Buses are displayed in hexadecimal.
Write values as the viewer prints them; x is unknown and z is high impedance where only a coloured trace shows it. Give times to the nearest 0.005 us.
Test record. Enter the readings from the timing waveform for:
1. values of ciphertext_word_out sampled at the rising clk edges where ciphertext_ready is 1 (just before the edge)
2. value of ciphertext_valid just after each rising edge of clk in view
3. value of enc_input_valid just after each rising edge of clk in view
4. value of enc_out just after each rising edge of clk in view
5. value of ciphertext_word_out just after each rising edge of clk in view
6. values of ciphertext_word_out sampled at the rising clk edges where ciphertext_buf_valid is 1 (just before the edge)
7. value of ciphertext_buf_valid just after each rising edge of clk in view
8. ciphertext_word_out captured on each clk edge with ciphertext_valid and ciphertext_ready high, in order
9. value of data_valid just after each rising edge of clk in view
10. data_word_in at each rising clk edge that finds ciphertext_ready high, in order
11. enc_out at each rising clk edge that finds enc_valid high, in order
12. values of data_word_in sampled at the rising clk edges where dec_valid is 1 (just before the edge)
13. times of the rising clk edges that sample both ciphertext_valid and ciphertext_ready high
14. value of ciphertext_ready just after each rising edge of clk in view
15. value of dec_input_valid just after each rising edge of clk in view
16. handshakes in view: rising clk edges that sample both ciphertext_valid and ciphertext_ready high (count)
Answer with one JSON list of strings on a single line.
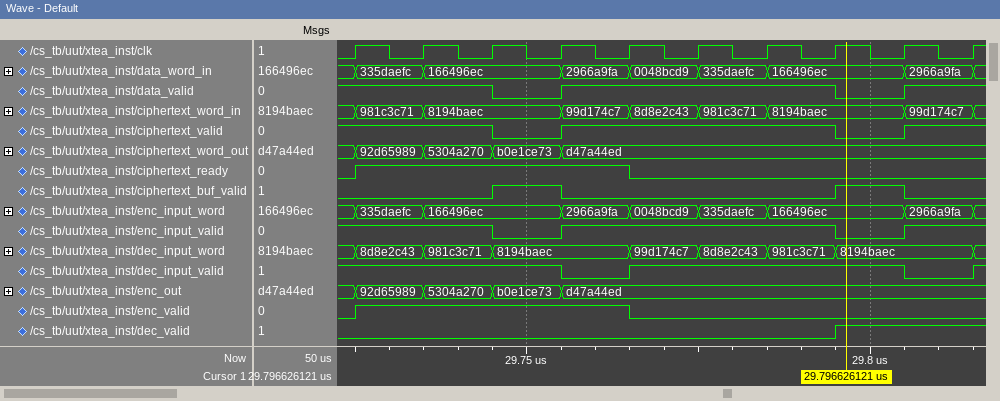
["92d65989, 5304a270, b0e1ce73, d47a44ed", "1 1 0 1 1 1 1 0 1 1", "1 1 0 1 1 1 1 0 1 1", "92d65989, 5304a270, b0e1ce73, d47a44ed, d47a44ed, d47a44ed, d47a44ed, d47a44ed, d47a44ed, d47a44ed", "92d65989, 5304a270, b0e1ce73, d47a44ed, d47a44ed, d47a44ed, d47a44ed, d47a44ed, d47a44ed, d47a44ed", "b0e1ce73, d47a44ed", "0 0 1 0 0 0 0 1 0 0", "92d65989, 5304a270, d47a44ed", "1 1 0 1 1 1 1 0 1 1", "335daefc, 166496ec, 166496ec, 2966a9fa", "92d65989, 5304a270, b0e1ce73, d47a44ed", "166496ec, 2966a9fa", "29.735 us, 29.745 us, 29.765 us", "1 1 1 1 0 0 0 0 0 0", "1 1 1 0 1 1 1 1 0 1", "3"]
